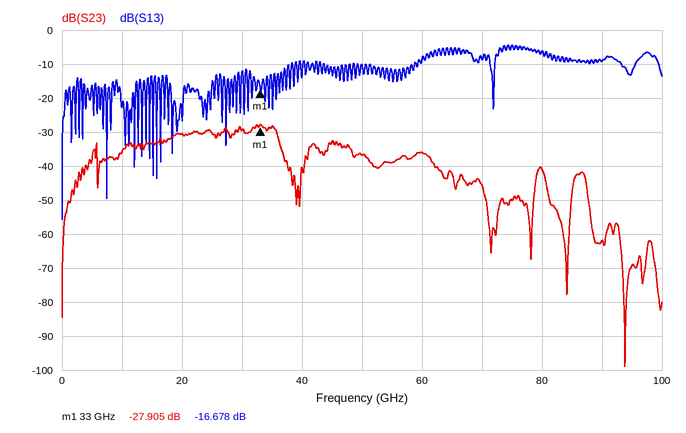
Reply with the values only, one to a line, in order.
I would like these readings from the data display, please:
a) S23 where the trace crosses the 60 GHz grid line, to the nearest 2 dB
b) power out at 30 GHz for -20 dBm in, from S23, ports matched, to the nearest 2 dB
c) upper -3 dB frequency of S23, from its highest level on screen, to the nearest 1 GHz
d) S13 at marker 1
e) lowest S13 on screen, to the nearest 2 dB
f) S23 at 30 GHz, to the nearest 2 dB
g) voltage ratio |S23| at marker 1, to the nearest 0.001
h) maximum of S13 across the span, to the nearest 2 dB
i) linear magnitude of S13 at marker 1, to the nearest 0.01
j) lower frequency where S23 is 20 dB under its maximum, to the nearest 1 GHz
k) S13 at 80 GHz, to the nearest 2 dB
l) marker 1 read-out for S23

-36 dB
-50 dBm
36 GHz
-16.678 dB
-56 dB
-30 dB
0.040
-4 dB
0.15
2 GHz
-6 dB
-27.905 dB
